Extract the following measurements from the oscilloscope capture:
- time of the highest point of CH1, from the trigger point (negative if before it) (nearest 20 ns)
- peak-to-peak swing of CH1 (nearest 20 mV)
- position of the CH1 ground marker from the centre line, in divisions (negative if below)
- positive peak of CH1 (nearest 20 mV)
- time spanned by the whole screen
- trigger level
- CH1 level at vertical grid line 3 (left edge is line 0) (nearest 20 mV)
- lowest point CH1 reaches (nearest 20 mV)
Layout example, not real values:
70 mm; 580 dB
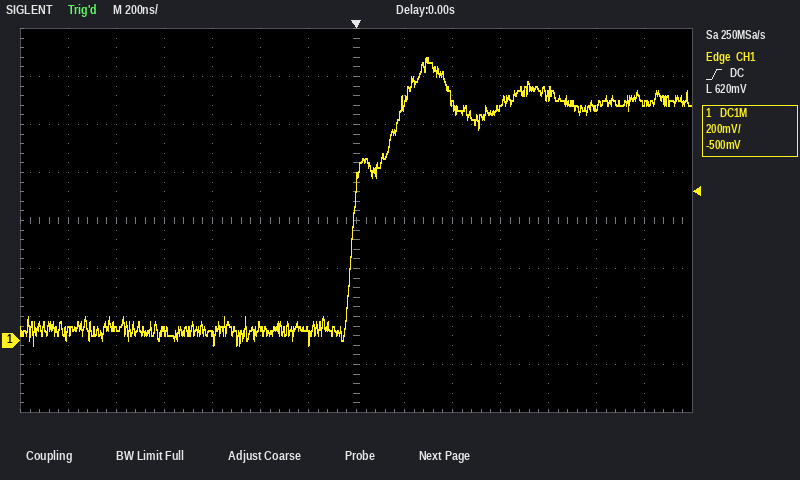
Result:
+300 ns; 1.20 V; -2.5 div; 1.18 V; 2.8 µs; 620 mV; 40 mV; -20 mV
